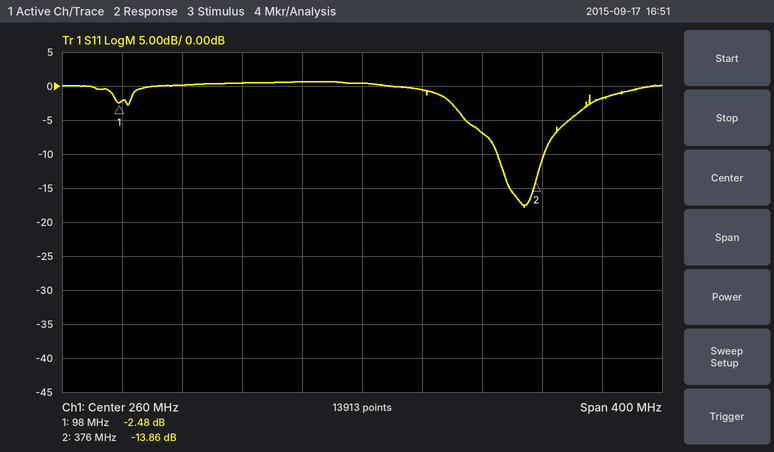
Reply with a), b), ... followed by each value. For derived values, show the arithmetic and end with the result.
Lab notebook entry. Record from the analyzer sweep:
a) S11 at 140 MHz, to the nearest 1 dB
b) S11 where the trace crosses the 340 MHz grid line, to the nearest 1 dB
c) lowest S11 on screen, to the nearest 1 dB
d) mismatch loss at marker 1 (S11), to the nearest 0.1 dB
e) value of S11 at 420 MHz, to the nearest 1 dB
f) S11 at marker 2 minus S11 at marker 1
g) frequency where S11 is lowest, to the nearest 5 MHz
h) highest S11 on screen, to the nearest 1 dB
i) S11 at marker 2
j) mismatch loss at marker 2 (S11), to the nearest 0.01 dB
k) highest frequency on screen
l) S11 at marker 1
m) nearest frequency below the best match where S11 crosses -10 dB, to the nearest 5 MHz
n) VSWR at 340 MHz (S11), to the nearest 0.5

a) 0 dB
b) -7 dB
c) -18 dB
d) −10 log10(1 − 10^(-2.48/10)) ≈ 3.6 dB
e) -2 dB
f) -13.86 − (-2.48) = -11.38 dB
g) 370 MHz
h) 1 dB
i) -13.86 dB
j) −10 log10(1 − 10^(-13.86/10)) ≈ 0.18 dB
k) 460 MHz
l) -2.48 dB
m) 350 MHz
n) |Γ| = 10^(-7/20) = 0.4467; VSWR = (1 + 0.4467)/(1 − 0.4467) ≈ 2.61, so 2.5 to the nearest 0.5
